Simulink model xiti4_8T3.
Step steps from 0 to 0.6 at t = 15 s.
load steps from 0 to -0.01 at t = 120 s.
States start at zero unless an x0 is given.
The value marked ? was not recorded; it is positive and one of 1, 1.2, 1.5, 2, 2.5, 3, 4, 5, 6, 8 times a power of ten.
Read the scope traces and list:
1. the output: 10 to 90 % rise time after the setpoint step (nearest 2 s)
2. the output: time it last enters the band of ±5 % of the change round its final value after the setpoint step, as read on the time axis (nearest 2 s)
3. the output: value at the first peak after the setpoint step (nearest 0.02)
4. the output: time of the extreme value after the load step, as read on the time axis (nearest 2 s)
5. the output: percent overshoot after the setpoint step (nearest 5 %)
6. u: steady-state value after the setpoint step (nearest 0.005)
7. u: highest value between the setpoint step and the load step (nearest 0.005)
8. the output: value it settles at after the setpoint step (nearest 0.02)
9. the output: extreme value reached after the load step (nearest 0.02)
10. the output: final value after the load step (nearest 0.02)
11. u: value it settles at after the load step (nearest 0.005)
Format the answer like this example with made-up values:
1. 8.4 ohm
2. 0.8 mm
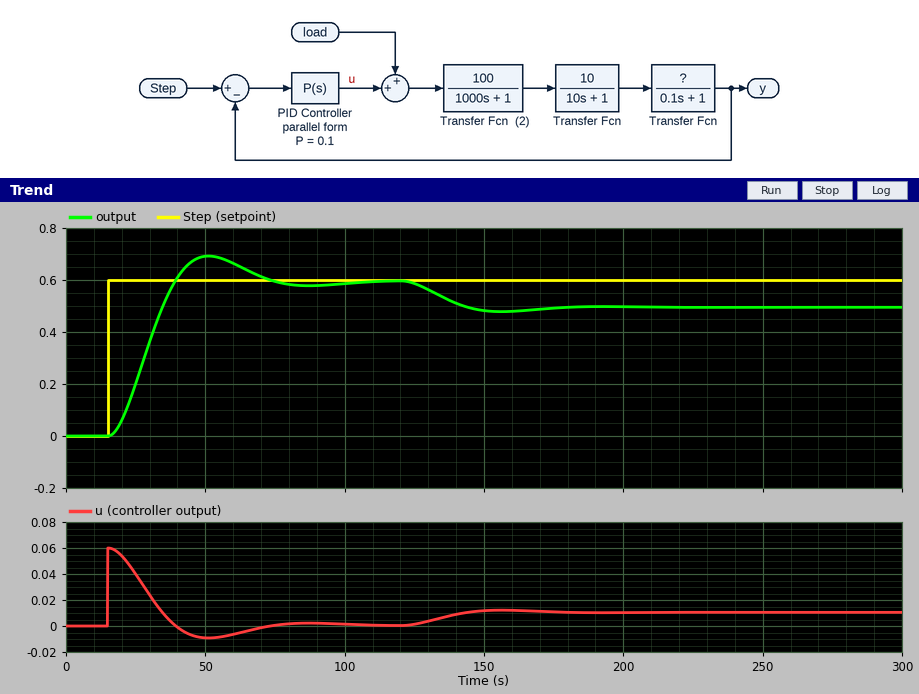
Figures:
1. 16 s
2. 68 s
3. 0.70
4. 156 s
5. 15 %
6. 0.000
7. 0.060
8. 0.60
9. 0.48
10. 0.50
11. 0.010
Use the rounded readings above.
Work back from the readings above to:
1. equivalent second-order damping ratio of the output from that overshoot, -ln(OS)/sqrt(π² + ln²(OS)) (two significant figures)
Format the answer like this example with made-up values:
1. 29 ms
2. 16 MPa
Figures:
1. 0.52
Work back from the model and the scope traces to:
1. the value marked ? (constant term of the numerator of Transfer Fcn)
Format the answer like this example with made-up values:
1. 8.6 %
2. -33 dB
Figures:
1. 1
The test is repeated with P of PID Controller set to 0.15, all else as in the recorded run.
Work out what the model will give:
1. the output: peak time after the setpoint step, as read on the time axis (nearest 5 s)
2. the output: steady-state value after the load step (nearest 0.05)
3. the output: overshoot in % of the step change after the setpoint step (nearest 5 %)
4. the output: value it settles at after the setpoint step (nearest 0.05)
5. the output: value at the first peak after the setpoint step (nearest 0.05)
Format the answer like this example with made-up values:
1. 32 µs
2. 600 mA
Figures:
1. 45 s
2. 0.55
3. 25 %
4. 0.60
5. 0.75
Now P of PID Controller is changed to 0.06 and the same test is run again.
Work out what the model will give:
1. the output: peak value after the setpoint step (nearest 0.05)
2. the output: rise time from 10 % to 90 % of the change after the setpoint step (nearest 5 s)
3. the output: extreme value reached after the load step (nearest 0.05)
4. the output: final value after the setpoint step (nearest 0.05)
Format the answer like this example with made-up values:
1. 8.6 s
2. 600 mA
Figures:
1. 0.65
2. 25 s
3. 0.40
4. 0.60
